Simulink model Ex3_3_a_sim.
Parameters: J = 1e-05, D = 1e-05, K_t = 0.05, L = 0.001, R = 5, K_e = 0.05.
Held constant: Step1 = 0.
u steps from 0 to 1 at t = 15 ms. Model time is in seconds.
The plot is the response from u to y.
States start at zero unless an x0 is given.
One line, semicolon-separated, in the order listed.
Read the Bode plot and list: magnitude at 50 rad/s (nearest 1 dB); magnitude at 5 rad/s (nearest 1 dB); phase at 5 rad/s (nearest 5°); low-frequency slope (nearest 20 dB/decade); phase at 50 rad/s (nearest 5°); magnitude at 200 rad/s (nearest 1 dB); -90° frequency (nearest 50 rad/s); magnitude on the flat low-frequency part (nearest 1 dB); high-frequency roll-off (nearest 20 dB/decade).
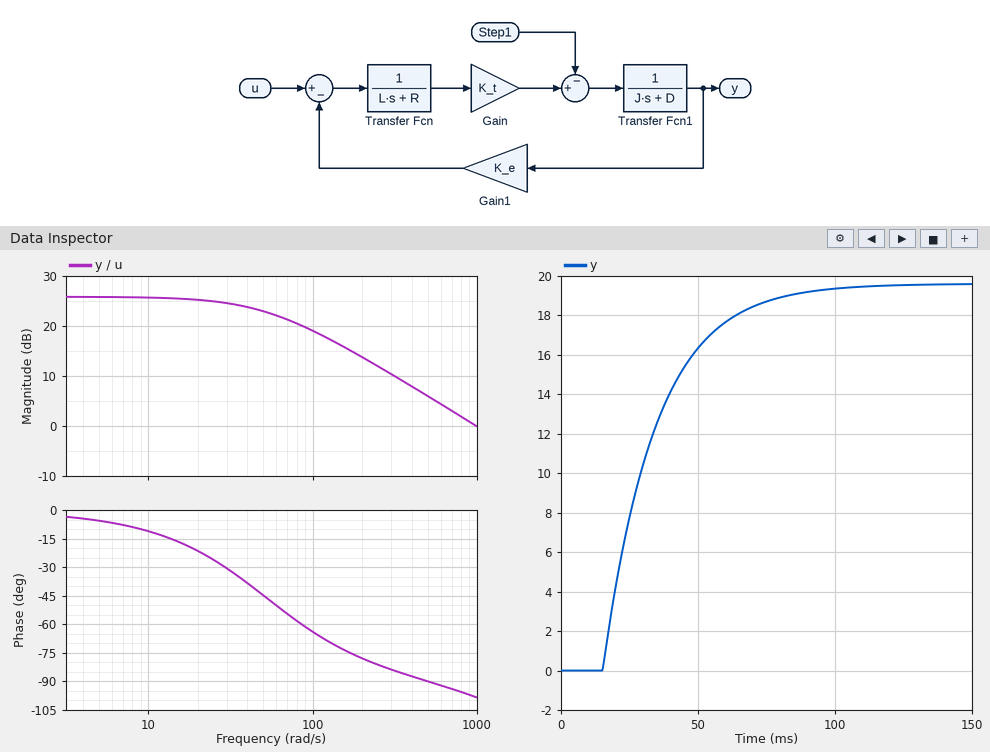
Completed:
23 dB; 26 dB; -5°; 0 dB/decade; -45°; 14 dB; 500 rad/s; 26 dB; -20 dB/decade
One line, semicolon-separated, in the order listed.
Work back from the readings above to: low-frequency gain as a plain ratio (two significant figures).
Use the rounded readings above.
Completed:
20
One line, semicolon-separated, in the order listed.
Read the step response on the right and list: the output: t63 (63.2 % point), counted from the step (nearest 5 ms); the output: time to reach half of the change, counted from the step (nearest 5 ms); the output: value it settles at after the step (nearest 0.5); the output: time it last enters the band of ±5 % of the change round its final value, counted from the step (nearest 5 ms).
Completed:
20 ms; 15 ms; 19.5; 60 ms
